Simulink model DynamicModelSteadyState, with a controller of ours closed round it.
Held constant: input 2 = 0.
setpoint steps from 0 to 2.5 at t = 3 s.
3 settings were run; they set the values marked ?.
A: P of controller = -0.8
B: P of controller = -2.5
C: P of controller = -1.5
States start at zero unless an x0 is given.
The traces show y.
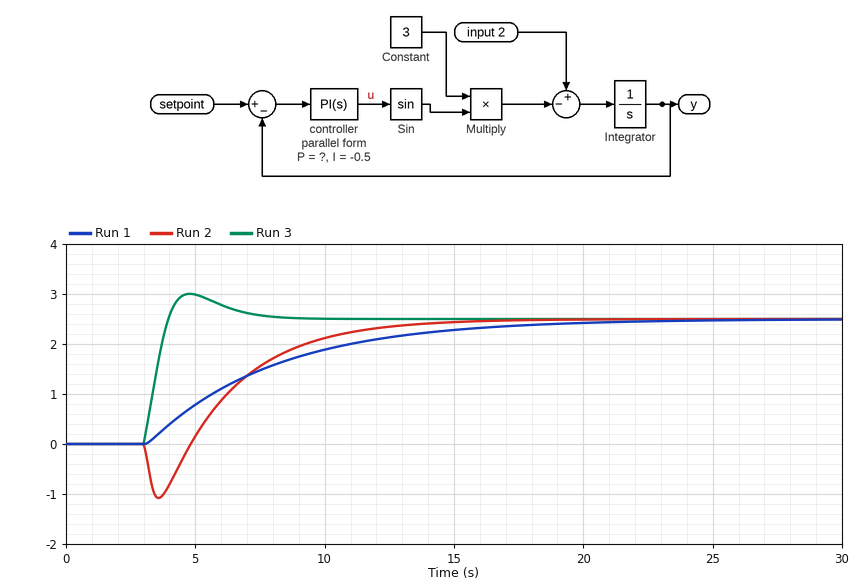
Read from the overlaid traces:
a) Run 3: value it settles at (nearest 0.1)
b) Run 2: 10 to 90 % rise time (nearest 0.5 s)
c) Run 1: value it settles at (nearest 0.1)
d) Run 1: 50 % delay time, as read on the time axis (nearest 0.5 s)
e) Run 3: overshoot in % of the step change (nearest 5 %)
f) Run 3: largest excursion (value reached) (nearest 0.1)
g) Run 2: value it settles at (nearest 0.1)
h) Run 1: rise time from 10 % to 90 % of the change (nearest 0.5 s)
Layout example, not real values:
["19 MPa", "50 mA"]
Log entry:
["2.5", "6.0 s", "2.5", "6.5 s", "20 %", "3.0", "2.5", "10.5 s"]
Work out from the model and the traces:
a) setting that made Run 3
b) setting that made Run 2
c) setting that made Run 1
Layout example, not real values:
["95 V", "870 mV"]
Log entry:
["A", "C", "B"]
